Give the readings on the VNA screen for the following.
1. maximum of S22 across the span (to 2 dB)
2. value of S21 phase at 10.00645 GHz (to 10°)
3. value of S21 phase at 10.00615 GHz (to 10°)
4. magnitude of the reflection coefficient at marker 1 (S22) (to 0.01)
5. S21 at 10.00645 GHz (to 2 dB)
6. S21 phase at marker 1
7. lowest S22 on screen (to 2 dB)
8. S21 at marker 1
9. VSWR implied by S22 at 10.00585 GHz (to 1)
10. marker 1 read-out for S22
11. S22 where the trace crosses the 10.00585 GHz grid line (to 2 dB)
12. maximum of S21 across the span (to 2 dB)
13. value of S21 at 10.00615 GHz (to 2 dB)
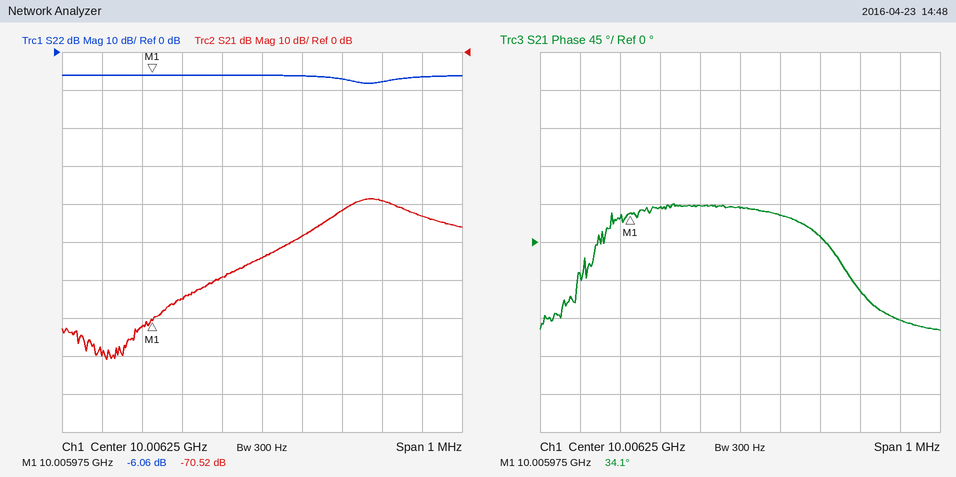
-6 dB
10°
40°
0.50
-42 dB
34.1°
-8 dB
-70.52 dB
3
-6.06 dB
-6 dB
-38 dB
-60 dB
